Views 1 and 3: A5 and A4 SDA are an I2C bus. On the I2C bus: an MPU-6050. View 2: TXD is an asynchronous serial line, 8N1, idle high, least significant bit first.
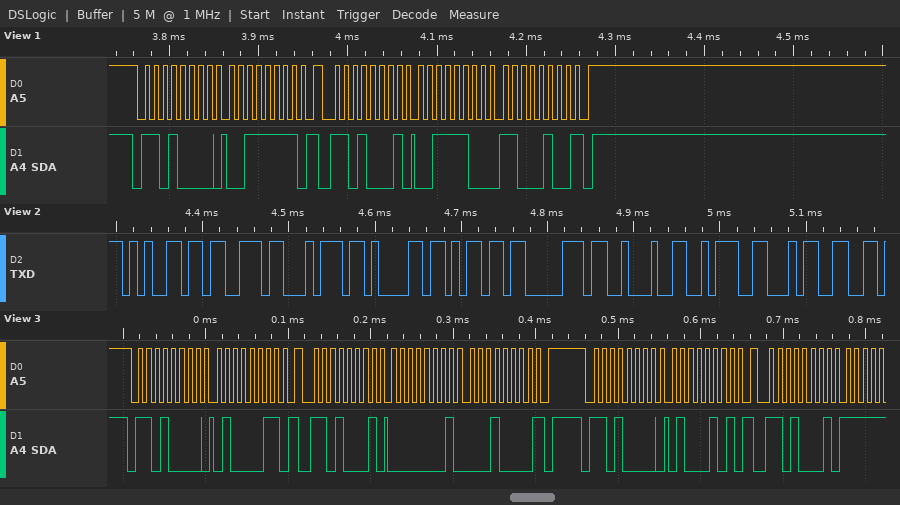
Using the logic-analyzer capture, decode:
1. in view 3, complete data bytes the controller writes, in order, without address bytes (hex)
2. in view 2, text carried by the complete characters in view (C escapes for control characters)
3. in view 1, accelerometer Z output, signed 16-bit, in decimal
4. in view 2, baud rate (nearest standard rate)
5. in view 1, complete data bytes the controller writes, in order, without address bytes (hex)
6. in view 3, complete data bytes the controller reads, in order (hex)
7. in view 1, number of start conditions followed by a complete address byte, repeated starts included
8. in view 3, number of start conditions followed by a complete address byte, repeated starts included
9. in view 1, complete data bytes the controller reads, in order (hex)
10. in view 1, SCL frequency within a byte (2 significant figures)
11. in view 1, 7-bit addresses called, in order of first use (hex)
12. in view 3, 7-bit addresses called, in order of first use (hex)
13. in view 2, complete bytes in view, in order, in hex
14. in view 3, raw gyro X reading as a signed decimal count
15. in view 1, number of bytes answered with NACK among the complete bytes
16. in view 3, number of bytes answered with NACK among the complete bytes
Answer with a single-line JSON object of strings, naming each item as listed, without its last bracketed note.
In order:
{"in view 3, complete data bytes the controller writes, in order, without address bytes": "43 45", "in view 2, text carried by the complete characters in view": "\"estamp\\\":4\"", "in view 1, accelerometer Z output, signed 16-bit, in decimal": "15556", "in view 2, baud rate": "115200 baud", "in view 1, complete data bytes the controller writes, in order, without address bytes": "3F", "in view 3, complete data bytes the controller reads, in order": "01 10", "in view 1, number of start conditions followed by a complete address byte, repeated starts included": "2", "in view 3, number of start conditions followed by a complete address byte, repeated starts included": "4", "in view 1, complete data bytes the controller reads, in order": "3C C4", "in view 1, SCL frequency within a byte": "100 kHz", "in view 1, 7-bit addresses called, in order of first use": "0x68", "in view 3, 7-bit addresses called, in order of first use": "0x68", "in view 2, complete bytes in view, in order, in hex": "65 73 74 61 6D 70 22 3A 34", "in view 3, raw gyro X reading as a signed decimal count": "272", "in view 1, number of bytes answered with NACK among the complete bytes": "1", "in view 3, number of bytes answered with NACK among the complete bytes": "1"}
